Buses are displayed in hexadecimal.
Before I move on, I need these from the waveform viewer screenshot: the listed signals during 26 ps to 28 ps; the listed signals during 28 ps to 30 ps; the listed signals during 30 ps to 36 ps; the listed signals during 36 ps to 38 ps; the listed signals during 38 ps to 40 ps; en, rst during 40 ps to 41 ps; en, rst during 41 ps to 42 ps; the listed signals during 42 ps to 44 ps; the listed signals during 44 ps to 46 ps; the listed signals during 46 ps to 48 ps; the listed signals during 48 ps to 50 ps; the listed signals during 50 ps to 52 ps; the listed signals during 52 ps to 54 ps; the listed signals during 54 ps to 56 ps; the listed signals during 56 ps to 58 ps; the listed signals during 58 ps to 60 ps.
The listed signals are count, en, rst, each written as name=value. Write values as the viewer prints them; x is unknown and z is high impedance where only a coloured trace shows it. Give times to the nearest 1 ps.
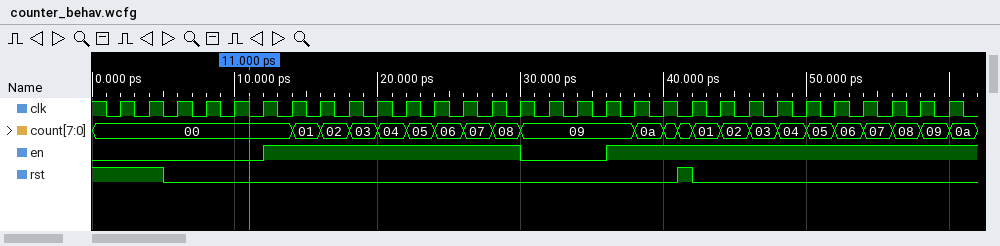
count=07, en=1, rst=0
count=08, en=1, rst=0
count=09, en=0, rst=0
count=09, en=1, rst=0
count=0a, en=1, rst=0
en=1, rst=0
en=1, rst=1
count=01, en=1, rst=0
count=02, en=1, rst=0
count=03, en=1, rst=0
count=04, en=1, rst=0
count=05, en=1, rst=0
count=06, en=1, rst=0
count=07, en=1, rst=0
count=08, en=1, rst=0
count=09, en=1, rst=0
